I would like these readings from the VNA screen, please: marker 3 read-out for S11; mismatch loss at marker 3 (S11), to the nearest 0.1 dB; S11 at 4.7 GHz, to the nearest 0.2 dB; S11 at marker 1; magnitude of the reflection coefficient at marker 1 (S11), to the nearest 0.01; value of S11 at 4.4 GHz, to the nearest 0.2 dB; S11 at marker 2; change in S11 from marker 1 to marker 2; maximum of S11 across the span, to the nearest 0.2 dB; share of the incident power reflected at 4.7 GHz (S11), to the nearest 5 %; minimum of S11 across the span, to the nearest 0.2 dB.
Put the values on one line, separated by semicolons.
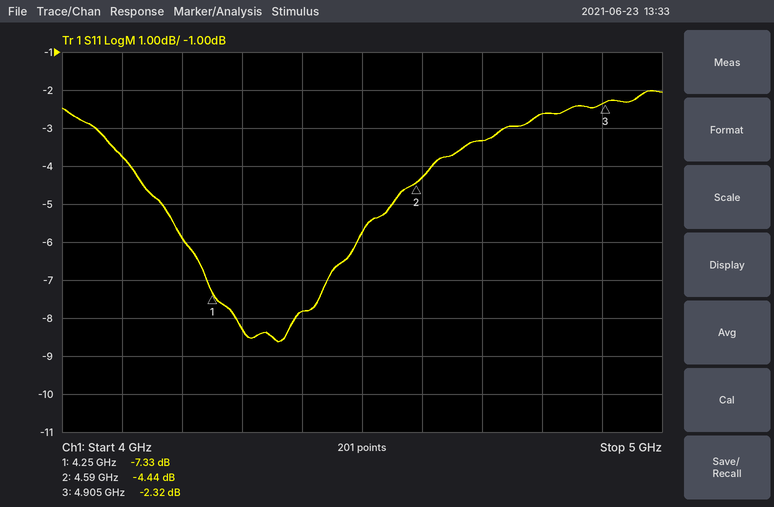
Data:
-2.32 dB; 3.8 dB; -3.4 dB; -7.33 dB; 0.43; -7.8 dB; -4.44 dB; 2.89 dB; -2.0 dB; 45 %; -8.6 dB
